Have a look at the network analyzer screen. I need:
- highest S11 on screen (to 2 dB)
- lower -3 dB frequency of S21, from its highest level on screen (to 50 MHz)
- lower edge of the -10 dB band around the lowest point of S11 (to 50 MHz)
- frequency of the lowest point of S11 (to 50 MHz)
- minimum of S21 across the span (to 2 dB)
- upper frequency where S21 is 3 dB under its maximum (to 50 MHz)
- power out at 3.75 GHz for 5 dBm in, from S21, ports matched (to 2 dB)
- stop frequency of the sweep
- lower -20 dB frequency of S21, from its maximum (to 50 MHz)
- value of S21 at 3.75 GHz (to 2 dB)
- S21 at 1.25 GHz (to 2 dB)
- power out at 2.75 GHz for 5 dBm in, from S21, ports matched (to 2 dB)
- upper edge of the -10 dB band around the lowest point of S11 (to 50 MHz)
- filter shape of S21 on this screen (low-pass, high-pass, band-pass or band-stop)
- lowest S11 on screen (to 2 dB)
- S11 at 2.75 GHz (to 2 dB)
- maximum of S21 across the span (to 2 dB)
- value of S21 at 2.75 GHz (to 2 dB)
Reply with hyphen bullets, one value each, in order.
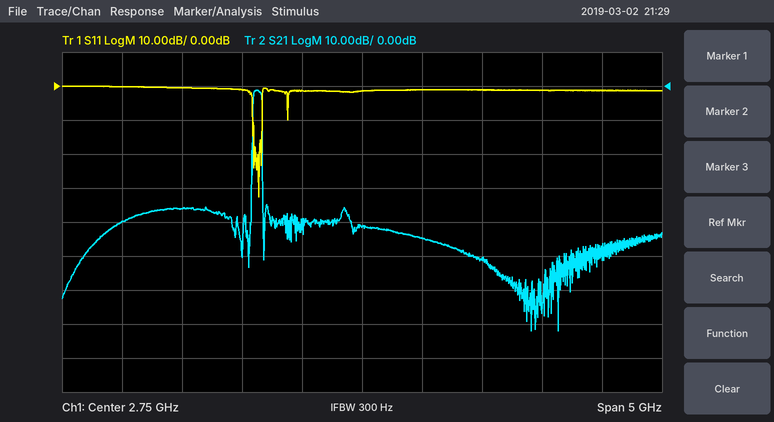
- 0 dB
- 1.85 GHz
- 1.85 GHz
- 1.90 GHz
- -72 dB
- 1.90 GHz
- -46 dBm
- 5.25 GHz
- 1.85 GHz
- -50 dB
- -36 dB
- -36 dBm
- 1.90 GHz
- band-pass
- -32 dB
- -2 dB
- -2 dB
- -42 dB
